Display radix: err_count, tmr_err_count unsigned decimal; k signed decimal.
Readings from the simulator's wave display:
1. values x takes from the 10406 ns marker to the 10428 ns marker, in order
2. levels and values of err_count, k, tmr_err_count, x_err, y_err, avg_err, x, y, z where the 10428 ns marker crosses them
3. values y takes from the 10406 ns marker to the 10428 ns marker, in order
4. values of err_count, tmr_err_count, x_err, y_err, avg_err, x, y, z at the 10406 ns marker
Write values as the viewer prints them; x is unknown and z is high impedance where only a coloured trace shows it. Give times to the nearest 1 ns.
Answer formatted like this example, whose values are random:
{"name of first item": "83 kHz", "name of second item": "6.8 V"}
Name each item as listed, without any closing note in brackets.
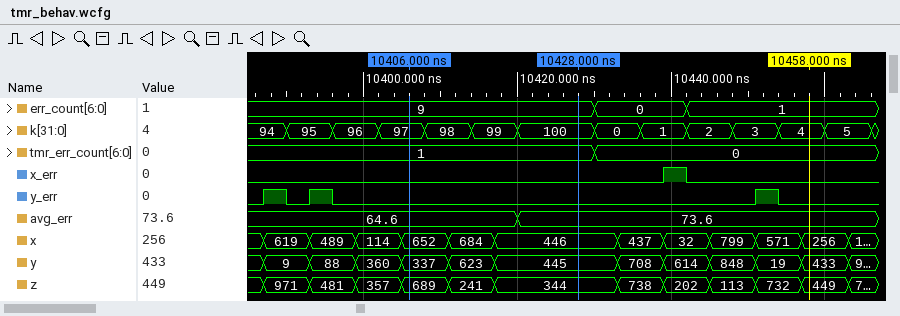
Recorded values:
{"values x takes from the 10406 ns marker to the 10428 ns marker, in order": "652, 684, 446", "levels and values of err_count, k, tmr_err_count, x_err, y_err, avg_err, x, y, z where the 10428 ns marker crosses them": "err_count=9, k=100, tmr_err_count=1, x_err=0, y_err=0, avg_err=73.6, x=446, y=445, z=344", "values y takes from the 10406 ns marker to the 10428 ns marker, in order": "337, 623, 445", "values of err_count, tmr_err_count, x_err, y_err, avg_err, x, y, z at the 10406 ns marker": "err_count=9, tmr_err_count=1, x_err=0, y_err=0, avg_err=64.6, x=652, y=337, z=689"}
